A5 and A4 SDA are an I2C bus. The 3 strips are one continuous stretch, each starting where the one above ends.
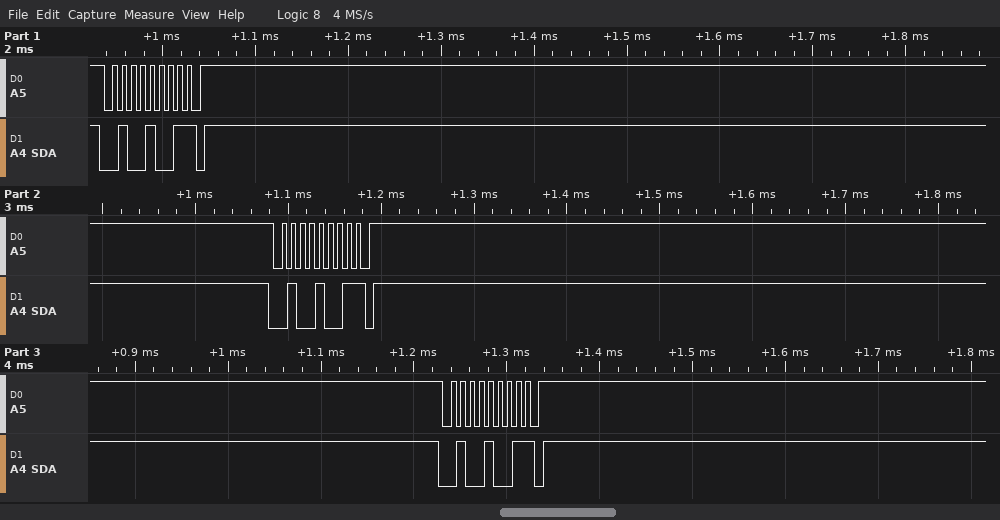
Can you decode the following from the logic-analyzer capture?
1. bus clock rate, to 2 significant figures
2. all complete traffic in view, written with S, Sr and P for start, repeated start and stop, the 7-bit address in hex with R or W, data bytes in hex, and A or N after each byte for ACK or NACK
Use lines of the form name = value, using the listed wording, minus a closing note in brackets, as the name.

bus clock rate, to 2 significant figures = 100 kHz
all complete traffic in view, written with S, Sr and P for start, repeated start and stop, the 7-bit address in hex with R or W, data bytes in hex, and A or N after each byte for ACK or NACK = S 24R N P S 24R N P S 24R N P
